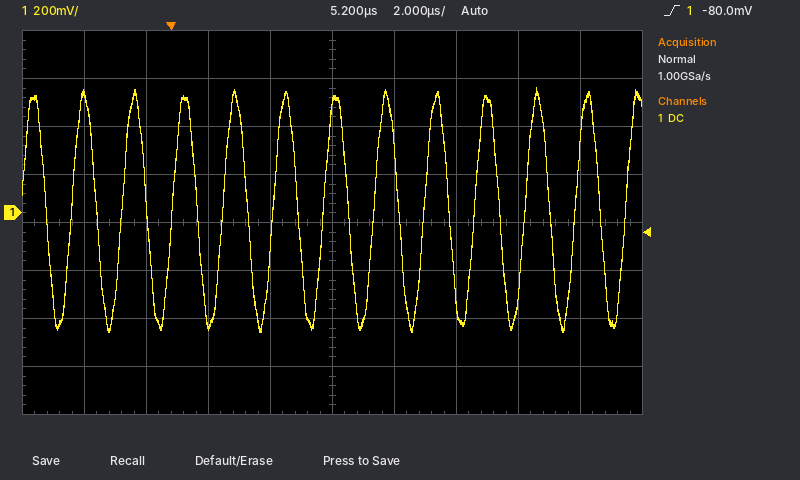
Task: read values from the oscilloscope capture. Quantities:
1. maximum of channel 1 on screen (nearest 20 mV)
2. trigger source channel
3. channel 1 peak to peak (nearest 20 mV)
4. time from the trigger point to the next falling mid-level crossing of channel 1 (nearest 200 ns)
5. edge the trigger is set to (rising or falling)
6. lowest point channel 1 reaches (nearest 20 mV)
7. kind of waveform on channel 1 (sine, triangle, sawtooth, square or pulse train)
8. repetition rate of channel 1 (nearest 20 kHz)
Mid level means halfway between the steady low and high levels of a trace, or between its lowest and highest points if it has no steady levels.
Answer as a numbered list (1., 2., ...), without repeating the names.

1. 520 mV
2. channel 1
3. 1.02 V
4. 800 ns
5. rising
6. -500 mV
7. sine
8. 620 kHz
